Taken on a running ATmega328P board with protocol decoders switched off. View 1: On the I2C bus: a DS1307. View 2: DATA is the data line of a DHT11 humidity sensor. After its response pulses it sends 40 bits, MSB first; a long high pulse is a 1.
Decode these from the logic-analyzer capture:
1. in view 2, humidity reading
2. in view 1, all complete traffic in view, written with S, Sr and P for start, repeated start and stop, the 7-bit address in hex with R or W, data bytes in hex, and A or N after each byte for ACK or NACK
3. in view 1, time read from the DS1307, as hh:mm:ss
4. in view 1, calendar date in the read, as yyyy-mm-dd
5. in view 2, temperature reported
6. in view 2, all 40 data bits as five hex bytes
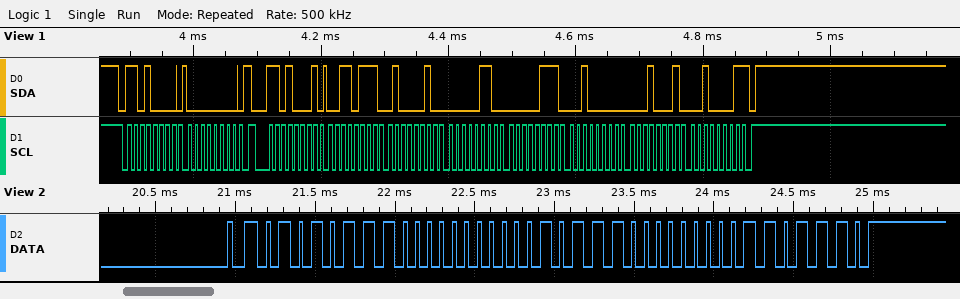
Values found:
87 %
S 68W A 00 A Sr 68R A 37 A 42 A 06 A 07 A 20 A 11 A 21 N P
06:42:37
2021-11-20
23.0 °C
57 00 17 00 6E
